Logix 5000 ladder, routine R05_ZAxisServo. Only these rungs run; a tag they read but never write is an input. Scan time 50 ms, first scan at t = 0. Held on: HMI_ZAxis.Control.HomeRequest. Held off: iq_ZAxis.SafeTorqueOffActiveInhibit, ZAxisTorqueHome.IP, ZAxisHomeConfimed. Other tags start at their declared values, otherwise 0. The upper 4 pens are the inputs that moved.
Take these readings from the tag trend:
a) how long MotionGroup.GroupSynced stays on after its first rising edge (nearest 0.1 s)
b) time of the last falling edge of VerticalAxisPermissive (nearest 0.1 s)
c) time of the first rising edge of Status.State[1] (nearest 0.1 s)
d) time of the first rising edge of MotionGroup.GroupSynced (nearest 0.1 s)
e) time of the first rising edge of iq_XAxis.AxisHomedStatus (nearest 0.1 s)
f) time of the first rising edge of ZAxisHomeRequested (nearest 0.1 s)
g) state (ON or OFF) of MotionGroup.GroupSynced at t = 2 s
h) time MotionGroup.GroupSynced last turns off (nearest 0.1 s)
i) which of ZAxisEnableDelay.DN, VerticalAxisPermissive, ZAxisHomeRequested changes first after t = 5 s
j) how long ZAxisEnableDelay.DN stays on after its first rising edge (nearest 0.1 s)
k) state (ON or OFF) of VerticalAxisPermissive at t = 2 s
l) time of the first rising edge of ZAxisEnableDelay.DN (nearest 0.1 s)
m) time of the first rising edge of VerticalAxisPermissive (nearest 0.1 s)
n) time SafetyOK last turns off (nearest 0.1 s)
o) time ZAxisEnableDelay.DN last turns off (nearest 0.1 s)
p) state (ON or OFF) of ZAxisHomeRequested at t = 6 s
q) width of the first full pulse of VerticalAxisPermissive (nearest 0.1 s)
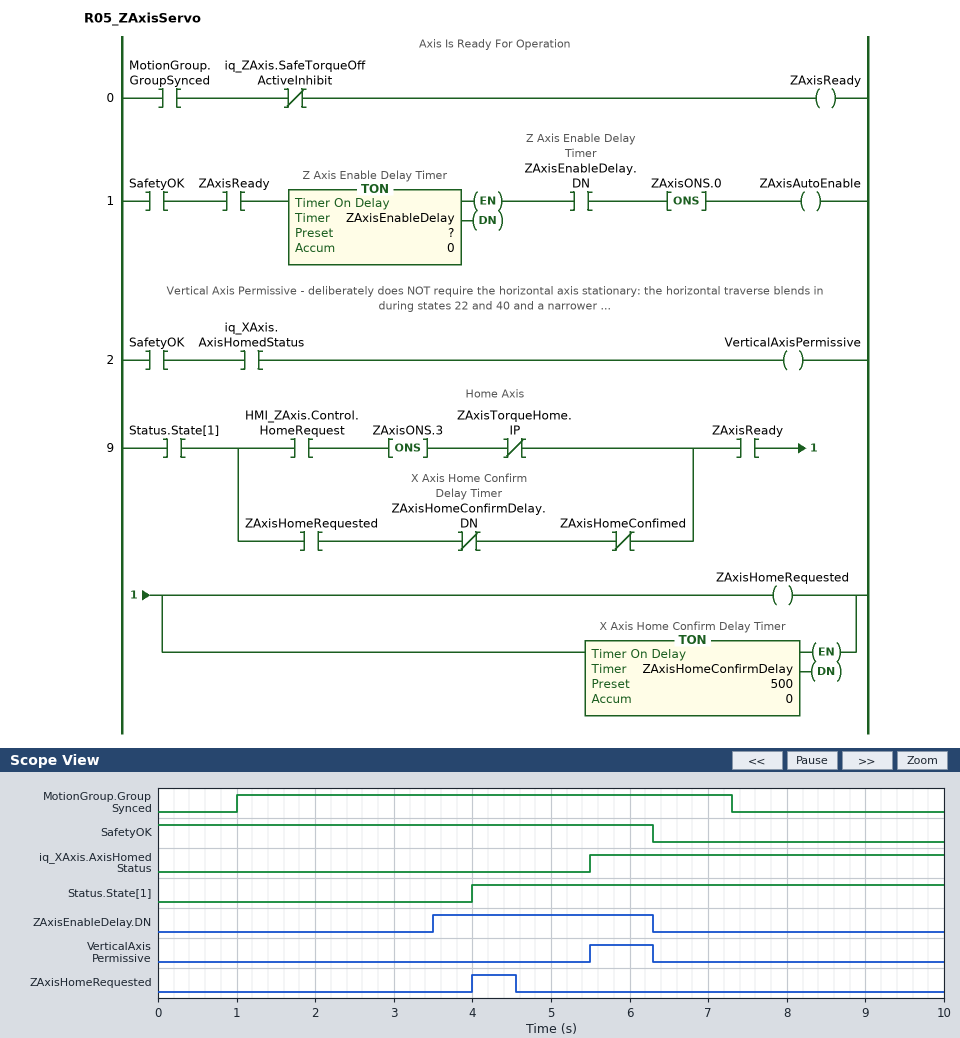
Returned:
6.3 s
6.3 s
4.0 s
1.0 s
5.5 s
4.0 s
ON
7.3 s
VerticalAxisPermissive
2.8 s
OFF
3.5 s
5.5 s
6.3 s
6.3 s
OFF
0.8 s
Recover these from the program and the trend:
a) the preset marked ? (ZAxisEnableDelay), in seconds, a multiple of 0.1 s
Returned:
2.5 s
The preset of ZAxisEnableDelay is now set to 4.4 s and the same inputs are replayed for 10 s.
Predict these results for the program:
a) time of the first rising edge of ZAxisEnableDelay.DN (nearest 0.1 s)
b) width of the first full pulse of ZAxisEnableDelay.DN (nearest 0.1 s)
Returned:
5.4 s
0.9 s
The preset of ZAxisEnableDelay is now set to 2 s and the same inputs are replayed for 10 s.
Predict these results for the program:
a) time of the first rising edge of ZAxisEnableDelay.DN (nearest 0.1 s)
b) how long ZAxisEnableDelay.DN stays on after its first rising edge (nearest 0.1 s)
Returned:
3.0 s
3.3 s
